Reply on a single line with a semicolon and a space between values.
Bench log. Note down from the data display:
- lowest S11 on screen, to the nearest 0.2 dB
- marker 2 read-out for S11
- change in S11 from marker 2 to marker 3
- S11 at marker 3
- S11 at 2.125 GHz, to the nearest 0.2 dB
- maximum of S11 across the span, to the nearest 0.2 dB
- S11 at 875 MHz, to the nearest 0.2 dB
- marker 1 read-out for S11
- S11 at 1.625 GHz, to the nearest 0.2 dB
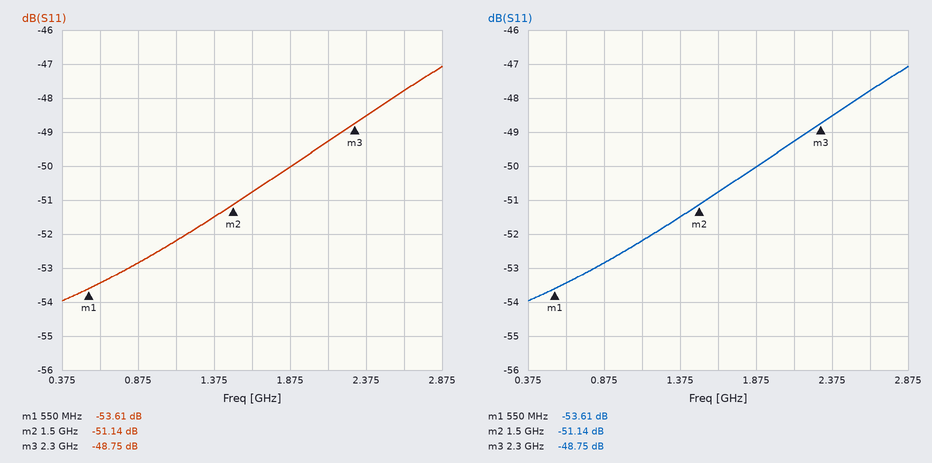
-54.0 dB; -51.14 dB; 2.39 dB; -48.75 dB; -49.2 dB; -47.0 dB; -52.8 dB; -53.61 dB; -50.8 dB
